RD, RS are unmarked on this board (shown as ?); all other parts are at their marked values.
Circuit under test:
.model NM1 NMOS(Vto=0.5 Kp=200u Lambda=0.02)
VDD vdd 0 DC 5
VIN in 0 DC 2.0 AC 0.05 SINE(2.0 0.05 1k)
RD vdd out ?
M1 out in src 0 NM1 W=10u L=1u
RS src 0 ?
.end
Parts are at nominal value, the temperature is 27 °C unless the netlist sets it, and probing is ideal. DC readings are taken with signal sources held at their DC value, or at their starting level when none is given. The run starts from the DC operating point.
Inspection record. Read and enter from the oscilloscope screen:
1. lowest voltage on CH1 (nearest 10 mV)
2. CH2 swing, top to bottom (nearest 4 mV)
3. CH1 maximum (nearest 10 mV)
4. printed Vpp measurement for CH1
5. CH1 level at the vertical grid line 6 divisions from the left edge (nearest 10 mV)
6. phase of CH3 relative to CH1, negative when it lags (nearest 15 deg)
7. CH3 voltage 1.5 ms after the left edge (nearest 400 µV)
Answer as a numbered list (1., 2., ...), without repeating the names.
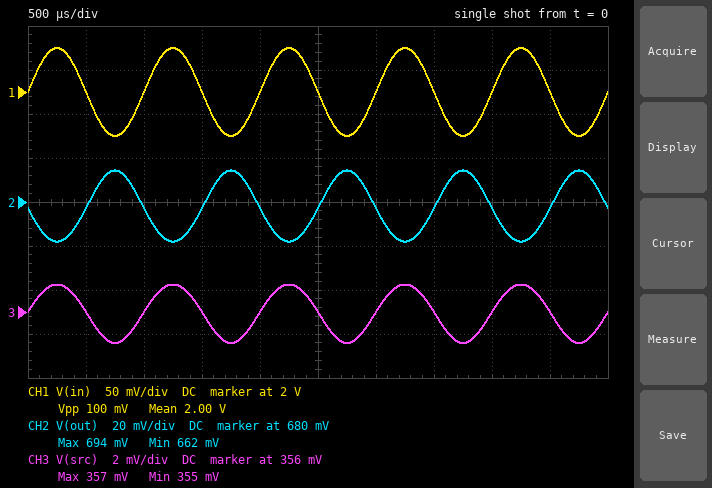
1. 1.95 V
2. 32 mV
3. 2.05 V
4. 100 mV
5. 2.00 V
6. 0 deg
7. 356.0 mV
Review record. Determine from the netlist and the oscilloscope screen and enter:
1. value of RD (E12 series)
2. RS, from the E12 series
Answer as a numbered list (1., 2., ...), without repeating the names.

1. 6.8 kΩ
2. 560 Ω
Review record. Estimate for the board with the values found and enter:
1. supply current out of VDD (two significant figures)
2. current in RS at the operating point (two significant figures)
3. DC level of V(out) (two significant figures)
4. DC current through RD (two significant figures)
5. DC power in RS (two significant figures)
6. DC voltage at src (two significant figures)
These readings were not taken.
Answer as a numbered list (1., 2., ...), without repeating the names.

1. 640 µA
2. 640 µA
3. 680 mV
4. 640 µA
5. 230 µW
6. 360 mV
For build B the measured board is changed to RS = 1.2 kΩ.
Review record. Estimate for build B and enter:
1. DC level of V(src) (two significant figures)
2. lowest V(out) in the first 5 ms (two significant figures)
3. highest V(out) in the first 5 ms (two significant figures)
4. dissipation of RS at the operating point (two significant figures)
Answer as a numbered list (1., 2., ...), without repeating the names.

1. 680 mV
2. 1.1 V
3. 1.2 V
4. 380 µW
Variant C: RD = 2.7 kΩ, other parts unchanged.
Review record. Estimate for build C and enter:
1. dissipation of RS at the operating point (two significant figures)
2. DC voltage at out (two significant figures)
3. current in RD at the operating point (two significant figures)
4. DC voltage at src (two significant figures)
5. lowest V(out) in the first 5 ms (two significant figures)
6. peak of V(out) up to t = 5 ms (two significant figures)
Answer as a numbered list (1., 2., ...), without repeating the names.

1. 520 µW
2. 2.4 V
3. 960 µA
4. 540 mV
5. 2.3 V
6. 2.5 V
